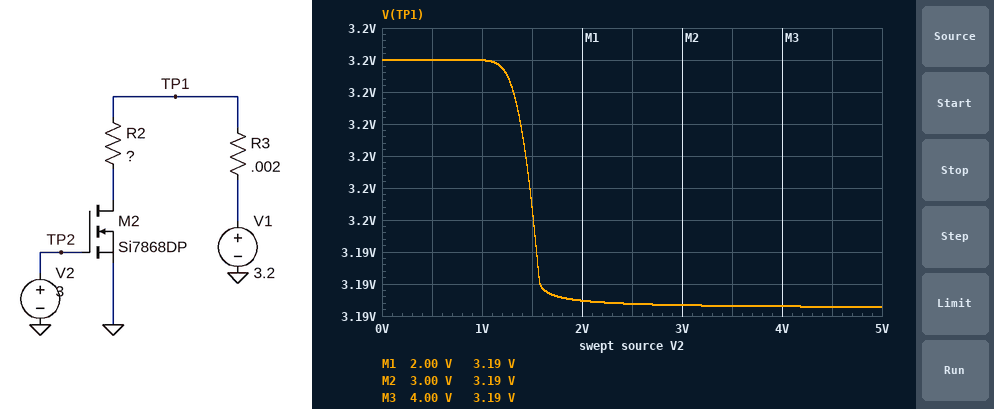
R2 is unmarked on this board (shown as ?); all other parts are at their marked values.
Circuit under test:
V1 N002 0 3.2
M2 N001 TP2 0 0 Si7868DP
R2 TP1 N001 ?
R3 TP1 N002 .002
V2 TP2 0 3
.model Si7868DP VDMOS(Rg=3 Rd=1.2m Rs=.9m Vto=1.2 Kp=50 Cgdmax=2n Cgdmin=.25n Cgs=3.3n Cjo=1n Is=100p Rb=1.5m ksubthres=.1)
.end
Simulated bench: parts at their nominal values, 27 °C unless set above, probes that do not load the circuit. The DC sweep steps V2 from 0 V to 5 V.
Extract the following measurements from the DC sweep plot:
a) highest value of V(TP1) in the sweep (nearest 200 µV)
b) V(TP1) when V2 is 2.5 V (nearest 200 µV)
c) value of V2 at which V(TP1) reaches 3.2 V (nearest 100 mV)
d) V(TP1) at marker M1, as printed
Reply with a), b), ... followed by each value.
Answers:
a) 3.2000 V
b) 3.1924 V
c) 1.5 V
d) 3.19 V
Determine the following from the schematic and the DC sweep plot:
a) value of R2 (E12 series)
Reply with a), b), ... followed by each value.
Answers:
a) 0.82 Ω
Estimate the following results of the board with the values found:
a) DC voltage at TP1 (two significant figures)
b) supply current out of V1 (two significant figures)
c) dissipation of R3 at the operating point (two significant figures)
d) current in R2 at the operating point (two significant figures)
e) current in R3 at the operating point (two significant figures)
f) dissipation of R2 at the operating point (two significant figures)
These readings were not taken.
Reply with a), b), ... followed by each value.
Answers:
a) 3.2 V
b) 3.8 A
c) 29 mW
d) 3.8 A
e) 3.8 A
f) 12 W
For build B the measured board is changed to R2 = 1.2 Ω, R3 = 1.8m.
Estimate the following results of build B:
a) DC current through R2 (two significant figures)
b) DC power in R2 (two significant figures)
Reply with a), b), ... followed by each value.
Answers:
a) 2.6 A
b) 8.3 W
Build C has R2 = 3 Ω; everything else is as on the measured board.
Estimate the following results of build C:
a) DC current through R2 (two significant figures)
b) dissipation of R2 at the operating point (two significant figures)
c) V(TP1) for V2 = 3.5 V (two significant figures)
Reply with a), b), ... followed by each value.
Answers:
a) 1.1 A
b) 3.4 W
c) 3.2 V
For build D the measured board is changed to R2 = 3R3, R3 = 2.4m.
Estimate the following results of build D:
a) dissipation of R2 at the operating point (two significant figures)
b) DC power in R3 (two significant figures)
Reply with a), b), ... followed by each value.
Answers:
a) 3.1 W
b) 2.2 mW
